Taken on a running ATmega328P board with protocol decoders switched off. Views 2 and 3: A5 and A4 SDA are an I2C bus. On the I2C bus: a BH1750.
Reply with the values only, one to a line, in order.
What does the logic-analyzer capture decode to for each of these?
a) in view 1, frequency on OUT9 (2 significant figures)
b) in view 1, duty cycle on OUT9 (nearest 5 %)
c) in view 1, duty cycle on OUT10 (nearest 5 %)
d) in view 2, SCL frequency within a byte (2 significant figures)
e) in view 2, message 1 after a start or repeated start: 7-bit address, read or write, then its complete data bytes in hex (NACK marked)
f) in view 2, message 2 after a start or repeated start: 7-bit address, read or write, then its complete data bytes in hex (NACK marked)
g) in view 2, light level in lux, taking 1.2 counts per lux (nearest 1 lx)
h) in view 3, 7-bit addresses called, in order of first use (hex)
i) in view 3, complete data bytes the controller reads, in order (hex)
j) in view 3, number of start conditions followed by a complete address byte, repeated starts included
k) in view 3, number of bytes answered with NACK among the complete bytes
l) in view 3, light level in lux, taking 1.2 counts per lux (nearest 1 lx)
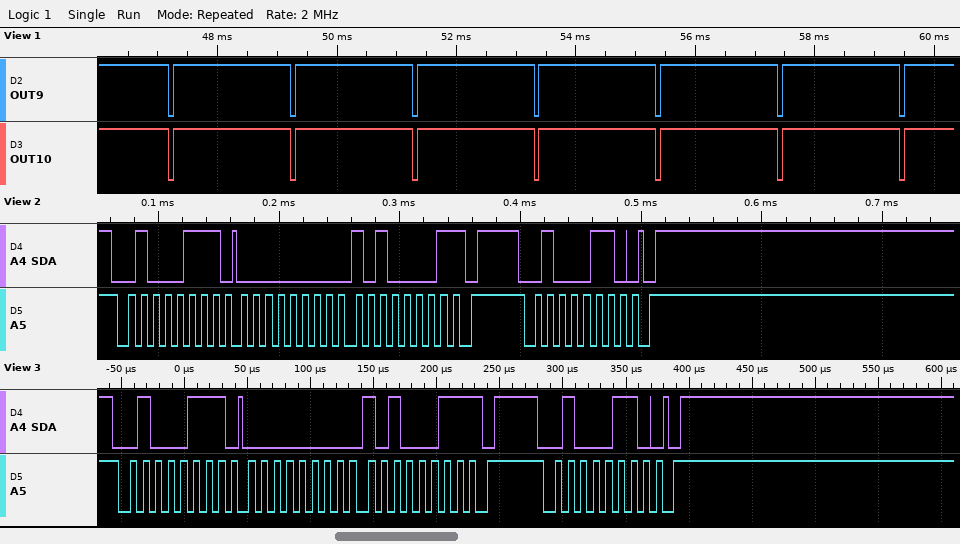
490 Hz
95 %
95 %
100 kHz
0x23 read: 00 A1 NACK
0x23 write
134 lx
0x23
00 A3
2
1
136 lx
